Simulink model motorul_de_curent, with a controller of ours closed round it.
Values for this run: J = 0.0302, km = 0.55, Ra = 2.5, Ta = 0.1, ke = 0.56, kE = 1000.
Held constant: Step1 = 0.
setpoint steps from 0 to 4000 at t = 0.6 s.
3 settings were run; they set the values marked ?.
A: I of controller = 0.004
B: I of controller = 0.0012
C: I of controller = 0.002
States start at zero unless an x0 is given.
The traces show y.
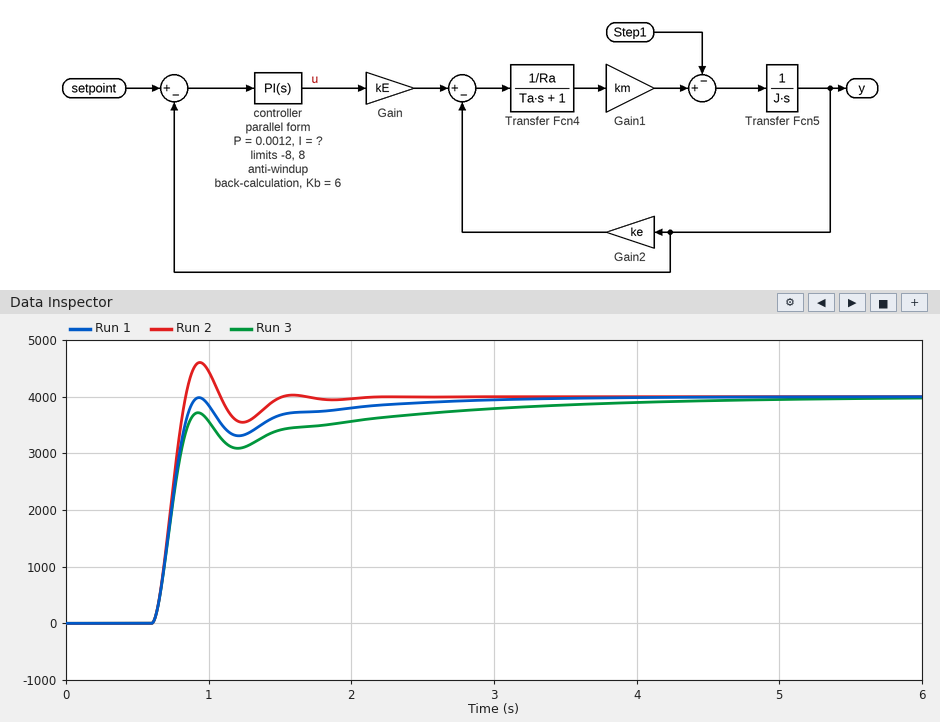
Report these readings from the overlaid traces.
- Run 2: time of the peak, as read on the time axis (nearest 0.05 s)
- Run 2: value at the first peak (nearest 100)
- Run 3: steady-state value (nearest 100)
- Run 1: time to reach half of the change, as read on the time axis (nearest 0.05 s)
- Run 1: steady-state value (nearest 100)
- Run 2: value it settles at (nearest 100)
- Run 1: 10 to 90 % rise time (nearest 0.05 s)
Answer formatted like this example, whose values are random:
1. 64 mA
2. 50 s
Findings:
1. 0.95 s
2. 4600
3. 4000
4. 0.75 s
5. 4000
6. 4000
7. 0.20 s
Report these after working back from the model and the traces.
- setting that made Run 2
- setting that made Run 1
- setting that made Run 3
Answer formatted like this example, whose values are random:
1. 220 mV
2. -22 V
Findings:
1. A
2. C
3. B
